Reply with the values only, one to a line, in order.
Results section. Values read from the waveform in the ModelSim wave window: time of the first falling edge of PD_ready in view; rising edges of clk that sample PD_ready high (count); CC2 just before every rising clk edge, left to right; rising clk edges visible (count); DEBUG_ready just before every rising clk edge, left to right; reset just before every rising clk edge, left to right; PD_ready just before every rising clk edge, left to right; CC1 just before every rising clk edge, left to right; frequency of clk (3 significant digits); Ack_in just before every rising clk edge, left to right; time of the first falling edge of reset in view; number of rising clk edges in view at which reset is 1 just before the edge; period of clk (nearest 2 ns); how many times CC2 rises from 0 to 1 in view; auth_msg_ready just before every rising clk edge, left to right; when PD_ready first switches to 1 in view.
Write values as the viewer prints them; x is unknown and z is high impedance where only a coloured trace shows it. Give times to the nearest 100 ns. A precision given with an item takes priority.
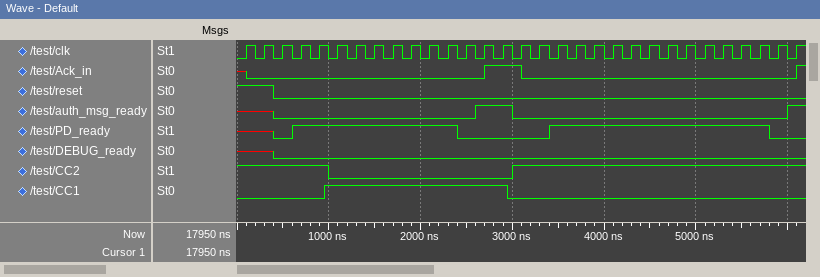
2400 ns
21
1 1 1 1 1 0 0 0 0 0 0 0 0 0 0 1 1 1 1 1 1 1 1 1 1 1 1 1 1 1 1
31
x x 0 0 0 0 0 0 0 0 0 0 0 0 0 0 0 0 0 0 0 0 0 0 0 0 0 0 0 0 0
1 1 0 0 0 0 0 0 0 0 0 0 0 0 0 0 0 0 0 0 0 0 0 0 0 0 0 0 0 0 0
x x 0 1 1 1 1 1 1 1 1 1 0 0 0 0 0 1 1 1 1 1 1 1 1 1 1 1 1 0 0
0 0 0 0 0 1 1 1 1 1 1 1 1 1 1 0 0 0 0 0 0 0 0 0 0 0 0 0 0 0 0
5.00 MHz
x 0 0 0 0 0 0 0 0 0 0 0 0 0 1 1 0 0 0 0 0 0 0 0 0 0 0 0 0 0 0
400 ns
2
200 ns
1
x x 0 0 0 0 0 0 0 0 0 0 0 1 1 0 0 0 0 0 0 0 0 0 0 0 0 0 0 0 1
600 ns
